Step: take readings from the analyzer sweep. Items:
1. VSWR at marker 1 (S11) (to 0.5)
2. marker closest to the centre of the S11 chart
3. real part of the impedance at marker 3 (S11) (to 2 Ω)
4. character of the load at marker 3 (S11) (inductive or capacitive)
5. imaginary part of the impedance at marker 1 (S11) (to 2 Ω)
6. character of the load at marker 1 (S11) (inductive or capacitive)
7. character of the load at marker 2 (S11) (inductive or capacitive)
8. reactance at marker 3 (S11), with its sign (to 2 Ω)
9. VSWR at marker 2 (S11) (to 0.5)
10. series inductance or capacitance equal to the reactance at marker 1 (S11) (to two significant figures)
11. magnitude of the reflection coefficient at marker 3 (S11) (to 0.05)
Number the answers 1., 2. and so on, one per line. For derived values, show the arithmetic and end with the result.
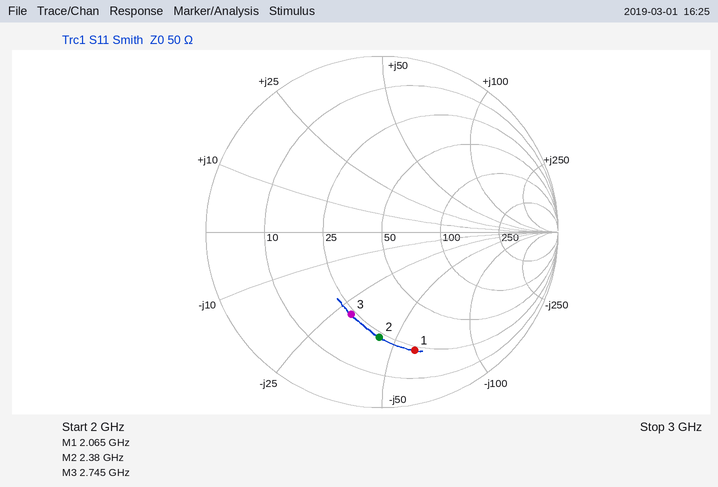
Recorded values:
1. 5.5
2. marker 3
3. 24 Ω
4. capacitive
5. -60 Ω
6. capacitive
7. capacitive
8. -30 Ω
9. 4.0
10. C = 1/(2π × 2.065 GHz × 60 Ω) ≈ 1.3 pF
11. 0.50
